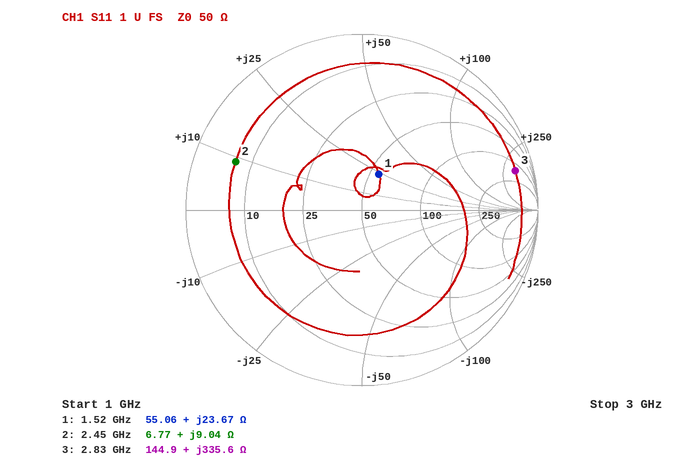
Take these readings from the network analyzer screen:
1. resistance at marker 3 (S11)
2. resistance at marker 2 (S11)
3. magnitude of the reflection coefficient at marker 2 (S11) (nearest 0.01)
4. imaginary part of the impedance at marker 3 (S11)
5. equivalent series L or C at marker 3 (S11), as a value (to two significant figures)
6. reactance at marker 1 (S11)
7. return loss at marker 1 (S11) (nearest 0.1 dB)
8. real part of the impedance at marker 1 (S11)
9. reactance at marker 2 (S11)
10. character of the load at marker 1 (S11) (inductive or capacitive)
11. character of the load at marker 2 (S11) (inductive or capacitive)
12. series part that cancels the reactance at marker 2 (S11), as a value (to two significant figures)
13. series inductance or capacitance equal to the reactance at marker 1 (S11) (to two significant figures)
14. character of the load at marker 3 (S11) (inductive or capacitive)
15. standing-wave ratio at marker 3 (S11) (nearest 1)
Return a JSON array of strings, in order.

["144.9 Ω", "6.77 Ω", "0.77", "+335.6 Ω", "19 nH", "+23.67 Ω", "13.0 dB", "55.06 Ω", "+9.04 Ω", "inductive", "inductive", "7.2 pF", "2.5 nH", "inductive", "19"]
